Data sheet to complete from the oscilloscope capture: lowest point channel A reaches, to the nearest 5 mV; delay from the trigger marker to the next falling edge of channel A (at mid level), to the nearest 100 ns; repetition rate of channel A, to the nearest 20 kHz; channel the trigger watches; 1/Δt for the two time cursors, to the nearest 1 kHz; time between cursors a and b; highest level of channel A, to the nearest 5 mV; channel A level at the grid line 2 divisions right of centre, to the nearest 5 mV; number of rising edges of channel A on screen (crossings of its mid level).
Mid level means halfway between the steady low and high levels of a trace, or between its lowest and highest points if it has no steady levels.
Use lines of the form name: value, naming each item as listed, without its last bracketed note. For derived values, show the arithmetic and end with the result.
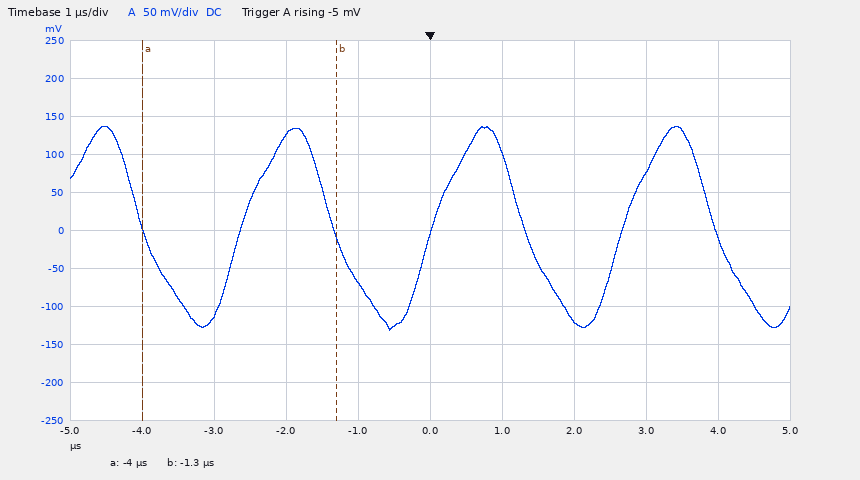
lowest point channel A reaches, to the nearest 5 mV: -130 mV
delay from the trigger marker to the next falling edge of channel A (at mid level), to the nearest 100 ns: 1.3 µs
repetition rate of channel A, to the nearest 20 kHz: 380 kHz
channel the trigger watches: channel A
1/Δt for the two time cursors, to the nearest 1 kHz: 1 / 2.7 µs ≈ 370 kHz
time between cursors a and b: -1.3 µs − (-4 µs) = 2.7 µs
highest level of channel A, to the nearest 5 mV: 135 mV
channel A level at the grid line 2 divisions right of centre, to the nearest 5 mV: -120 mV
number of rising edges of channel A on screen: 3
